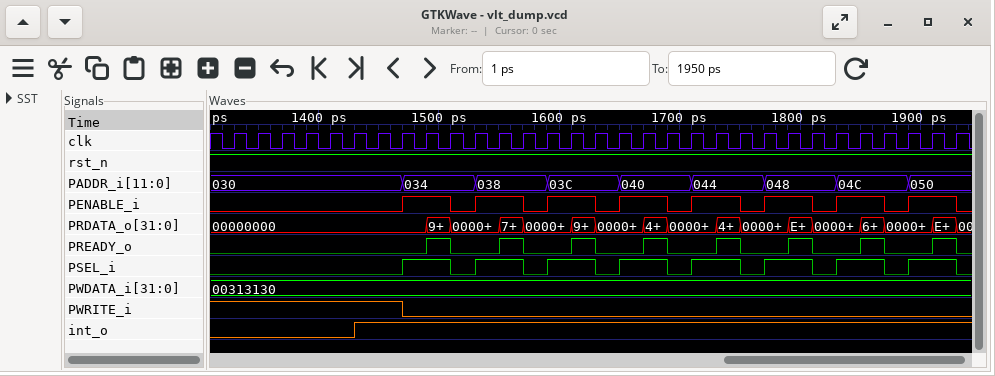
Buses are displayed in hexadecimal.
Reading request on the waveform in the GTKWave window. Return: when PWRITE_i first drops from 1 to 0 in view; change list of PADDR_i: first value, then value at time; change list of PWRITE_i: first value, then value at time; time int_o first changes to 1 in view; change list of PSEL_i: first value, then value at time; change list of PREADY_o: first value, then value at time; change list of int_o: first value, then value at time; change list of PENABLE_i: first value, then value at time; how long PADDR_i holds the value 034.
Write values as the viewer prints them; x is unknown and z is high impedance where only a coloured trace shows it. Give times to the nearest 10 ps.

1470 ps
030, 034 at 1470 ps, 038 at 1530 ps, 03C at 1590 ps, 040 at 1650 ps, 044 at 1710 ps, 048 at 1770 ps, 04C at 1830 ps, 050 at 1890 ps
1, 0 at 1470 ps
1430 ps
0, 1 at 1470 ps, 0 at 1510 ps, 1 at 1530 ps, 0 at 1570 ps, 1 at 1590 ps, 0 at 1630 ps, 1 at 1650 ps, 0 at 1690 ps, 1 at 1710 ps, 0 at 1750 ps, 1 at 1770 ps, 0 at 1810 ps, 1 at 1830 ps, 0 at 1870 ps, 1 at 1890 ps, 0 at 1930 ps
0, 1 at 1490 ps, 0 at 1510 ps, 1 at 1550 ps, 0 at 1570 ps, 1 at 1610 ps, 0 at 1630 ps, 1 at 1670 ps, 0 at 1690 ps, 1 at 1730 ps, 0 at 1750 ps, 1 at 1790 ps, 0 at 1810 ps, 1 at 1850 ps, 0 at 1870 ps, 1 at 1910 ps, 0 at 1930 ps
0, 1 at 1430 ps
0, 1 at 1470 ps, 0 at 1510 ps, 1 at 1530 ps, 0 at 1570 ps, 1 at 1590 ps, 0 at 1630 ps, 1 at 1650 ps, 0 at 1690 ps, 1 at 1710 ps, 0 at 1750 ps, 1 at 1770 ps, 0 at 1810 ps, 1 at 1830 ps, 0 at 1870 ps, 1 at 1890 ps, 0 at 1930 ps
60 ps
